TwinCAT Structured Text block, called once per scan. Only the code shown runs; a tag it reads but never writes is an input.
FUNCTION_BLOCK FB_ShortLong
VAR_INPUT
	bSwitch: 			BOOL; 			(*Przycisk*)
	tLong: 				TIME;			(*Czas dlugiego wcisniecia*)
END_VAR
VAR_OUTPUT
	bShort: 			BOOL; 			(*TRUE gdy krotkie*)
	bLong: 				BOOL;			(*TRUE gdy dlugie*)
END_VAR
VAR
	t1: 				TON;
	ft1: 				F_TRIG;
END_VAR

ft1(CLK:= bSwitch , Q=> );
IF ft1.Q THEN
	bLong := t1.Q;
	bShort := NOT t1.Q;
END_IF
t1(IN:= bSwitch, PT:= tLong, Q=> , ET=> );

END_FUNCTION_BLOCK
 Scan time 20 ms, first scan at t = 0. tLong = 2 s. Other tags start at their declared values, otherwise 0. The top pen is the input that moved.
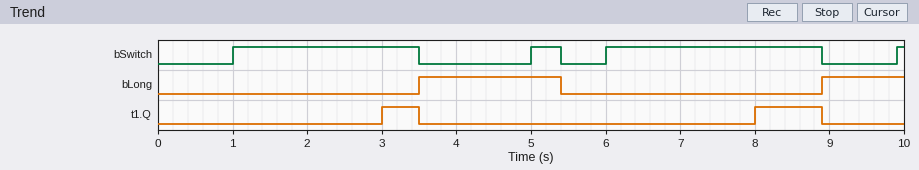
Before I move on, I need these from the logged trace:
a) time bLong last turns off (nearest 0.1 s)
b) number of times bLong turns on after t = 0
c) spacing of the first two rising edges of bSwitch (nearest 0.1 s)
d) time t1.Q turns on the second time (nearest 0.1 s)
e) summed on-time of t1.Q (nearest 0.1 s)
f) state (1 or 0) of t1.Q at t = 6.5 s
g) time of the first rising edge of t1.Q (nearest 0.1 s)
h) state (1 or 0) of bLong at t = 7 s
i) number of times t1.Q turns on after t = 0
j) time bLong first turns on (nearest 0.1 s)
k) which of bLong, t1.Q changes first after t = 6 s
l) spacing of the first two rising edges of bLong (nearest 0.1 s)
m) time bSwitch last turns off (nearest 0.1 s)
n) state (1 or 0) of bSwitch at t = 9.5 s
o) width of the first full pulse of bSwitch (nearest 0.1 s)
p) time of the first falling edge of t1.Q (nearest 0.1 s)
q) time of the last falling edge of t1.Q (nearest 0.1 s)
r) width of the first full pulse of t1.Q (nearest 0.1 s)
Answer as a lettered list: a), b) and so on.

a) 5.4 s
b) 2
c) 4.0 s
d) 8.0 s
e) 1.4 s
f) 0
g) 3.0 s
h) 0
i) 2
j) 3.5 s
k) t1.Q
l) 5.4 s
m) 8.9 s
n) 0
o) 2.5 s
p) 3.5 s
q) 8.9 s
r) 0.5 s
